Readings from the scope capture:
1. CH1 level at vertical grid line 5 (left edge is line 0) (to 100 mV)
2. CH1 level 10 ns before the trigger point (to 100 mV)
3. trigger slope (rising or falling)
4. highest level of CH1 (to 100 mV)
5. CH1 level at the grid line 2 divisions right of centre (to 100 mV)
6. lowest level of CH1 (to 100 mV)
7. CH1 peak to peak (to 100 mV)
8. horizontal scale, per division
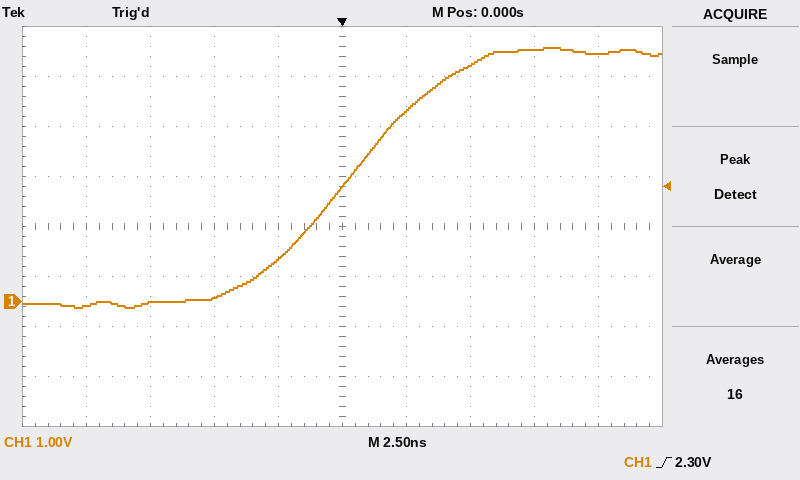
2.3 V
-100 mV
rising
5.1 V
4.7 V
-100 mV
5.2 V
2.5 ns
